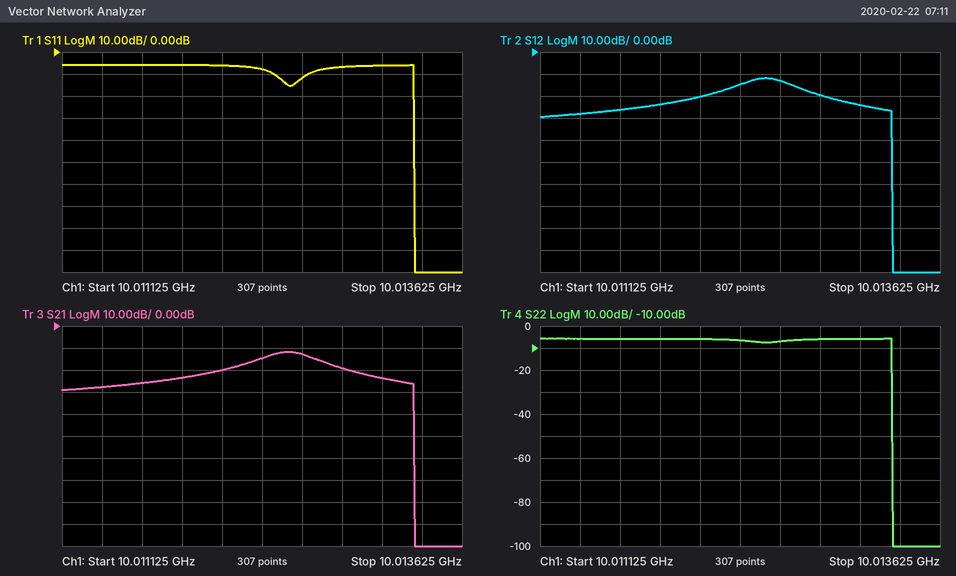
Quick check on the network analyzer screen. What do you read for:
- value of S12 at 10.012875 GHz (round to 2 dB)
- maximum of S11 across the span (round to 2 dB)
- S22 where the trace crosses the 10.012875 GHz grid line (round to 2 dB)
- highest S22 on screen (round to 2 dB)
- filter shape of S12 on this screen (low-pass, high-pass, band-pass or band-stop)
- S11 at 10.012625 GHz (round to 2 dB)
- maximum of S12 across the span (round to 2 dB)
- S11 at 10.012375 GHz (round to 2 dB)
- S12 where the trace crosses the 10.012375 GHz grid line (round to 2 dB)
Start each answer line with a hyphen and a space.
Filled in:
- -20 dB
- -6 dB
- -6 dB
- -6 dB
- band-pass
- -12 dB
- -12 dB
- -8 dB
- -14 dB
